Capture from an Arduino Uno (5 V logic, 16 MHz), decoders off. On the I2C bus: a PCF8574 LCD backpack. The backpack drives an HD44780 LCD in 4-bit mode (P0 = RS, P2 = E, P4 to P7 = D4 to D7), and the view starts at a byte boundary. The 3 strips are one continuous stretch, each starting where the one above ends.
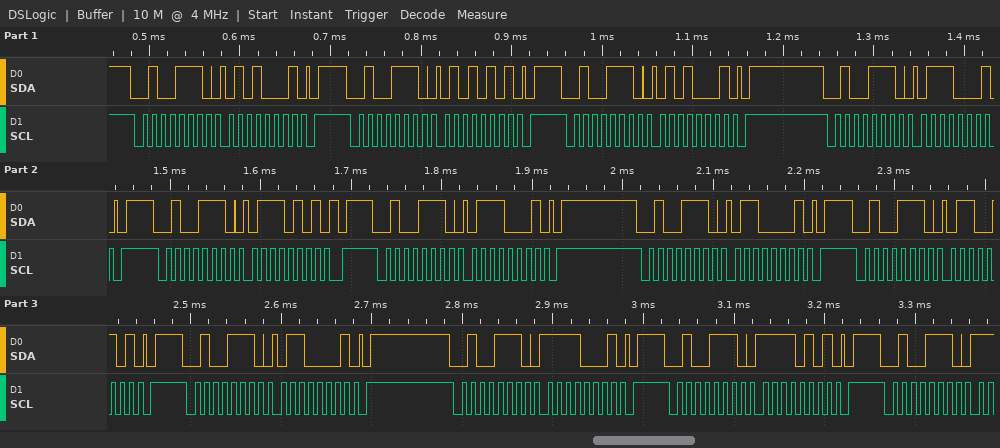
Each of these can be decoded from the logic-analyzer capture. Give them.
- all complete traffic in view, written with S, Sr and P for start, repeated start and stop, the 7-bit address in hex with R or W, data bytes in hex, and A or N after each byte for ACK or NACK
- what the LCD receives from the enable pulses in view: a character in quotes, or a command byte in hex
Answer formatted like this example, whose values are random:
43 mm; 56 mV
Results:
S 27W A 51 A P S 27W A 55 A P S 27W A 51 A P S 27W A 71 A P S 27W A 75 A P S 27W A 71 A P S 27W A 61 A P S 27W A 65 A P S 27W A 61 A P S 27W A F1 A P S 27W A F5 A P S 27W A; 'W'
